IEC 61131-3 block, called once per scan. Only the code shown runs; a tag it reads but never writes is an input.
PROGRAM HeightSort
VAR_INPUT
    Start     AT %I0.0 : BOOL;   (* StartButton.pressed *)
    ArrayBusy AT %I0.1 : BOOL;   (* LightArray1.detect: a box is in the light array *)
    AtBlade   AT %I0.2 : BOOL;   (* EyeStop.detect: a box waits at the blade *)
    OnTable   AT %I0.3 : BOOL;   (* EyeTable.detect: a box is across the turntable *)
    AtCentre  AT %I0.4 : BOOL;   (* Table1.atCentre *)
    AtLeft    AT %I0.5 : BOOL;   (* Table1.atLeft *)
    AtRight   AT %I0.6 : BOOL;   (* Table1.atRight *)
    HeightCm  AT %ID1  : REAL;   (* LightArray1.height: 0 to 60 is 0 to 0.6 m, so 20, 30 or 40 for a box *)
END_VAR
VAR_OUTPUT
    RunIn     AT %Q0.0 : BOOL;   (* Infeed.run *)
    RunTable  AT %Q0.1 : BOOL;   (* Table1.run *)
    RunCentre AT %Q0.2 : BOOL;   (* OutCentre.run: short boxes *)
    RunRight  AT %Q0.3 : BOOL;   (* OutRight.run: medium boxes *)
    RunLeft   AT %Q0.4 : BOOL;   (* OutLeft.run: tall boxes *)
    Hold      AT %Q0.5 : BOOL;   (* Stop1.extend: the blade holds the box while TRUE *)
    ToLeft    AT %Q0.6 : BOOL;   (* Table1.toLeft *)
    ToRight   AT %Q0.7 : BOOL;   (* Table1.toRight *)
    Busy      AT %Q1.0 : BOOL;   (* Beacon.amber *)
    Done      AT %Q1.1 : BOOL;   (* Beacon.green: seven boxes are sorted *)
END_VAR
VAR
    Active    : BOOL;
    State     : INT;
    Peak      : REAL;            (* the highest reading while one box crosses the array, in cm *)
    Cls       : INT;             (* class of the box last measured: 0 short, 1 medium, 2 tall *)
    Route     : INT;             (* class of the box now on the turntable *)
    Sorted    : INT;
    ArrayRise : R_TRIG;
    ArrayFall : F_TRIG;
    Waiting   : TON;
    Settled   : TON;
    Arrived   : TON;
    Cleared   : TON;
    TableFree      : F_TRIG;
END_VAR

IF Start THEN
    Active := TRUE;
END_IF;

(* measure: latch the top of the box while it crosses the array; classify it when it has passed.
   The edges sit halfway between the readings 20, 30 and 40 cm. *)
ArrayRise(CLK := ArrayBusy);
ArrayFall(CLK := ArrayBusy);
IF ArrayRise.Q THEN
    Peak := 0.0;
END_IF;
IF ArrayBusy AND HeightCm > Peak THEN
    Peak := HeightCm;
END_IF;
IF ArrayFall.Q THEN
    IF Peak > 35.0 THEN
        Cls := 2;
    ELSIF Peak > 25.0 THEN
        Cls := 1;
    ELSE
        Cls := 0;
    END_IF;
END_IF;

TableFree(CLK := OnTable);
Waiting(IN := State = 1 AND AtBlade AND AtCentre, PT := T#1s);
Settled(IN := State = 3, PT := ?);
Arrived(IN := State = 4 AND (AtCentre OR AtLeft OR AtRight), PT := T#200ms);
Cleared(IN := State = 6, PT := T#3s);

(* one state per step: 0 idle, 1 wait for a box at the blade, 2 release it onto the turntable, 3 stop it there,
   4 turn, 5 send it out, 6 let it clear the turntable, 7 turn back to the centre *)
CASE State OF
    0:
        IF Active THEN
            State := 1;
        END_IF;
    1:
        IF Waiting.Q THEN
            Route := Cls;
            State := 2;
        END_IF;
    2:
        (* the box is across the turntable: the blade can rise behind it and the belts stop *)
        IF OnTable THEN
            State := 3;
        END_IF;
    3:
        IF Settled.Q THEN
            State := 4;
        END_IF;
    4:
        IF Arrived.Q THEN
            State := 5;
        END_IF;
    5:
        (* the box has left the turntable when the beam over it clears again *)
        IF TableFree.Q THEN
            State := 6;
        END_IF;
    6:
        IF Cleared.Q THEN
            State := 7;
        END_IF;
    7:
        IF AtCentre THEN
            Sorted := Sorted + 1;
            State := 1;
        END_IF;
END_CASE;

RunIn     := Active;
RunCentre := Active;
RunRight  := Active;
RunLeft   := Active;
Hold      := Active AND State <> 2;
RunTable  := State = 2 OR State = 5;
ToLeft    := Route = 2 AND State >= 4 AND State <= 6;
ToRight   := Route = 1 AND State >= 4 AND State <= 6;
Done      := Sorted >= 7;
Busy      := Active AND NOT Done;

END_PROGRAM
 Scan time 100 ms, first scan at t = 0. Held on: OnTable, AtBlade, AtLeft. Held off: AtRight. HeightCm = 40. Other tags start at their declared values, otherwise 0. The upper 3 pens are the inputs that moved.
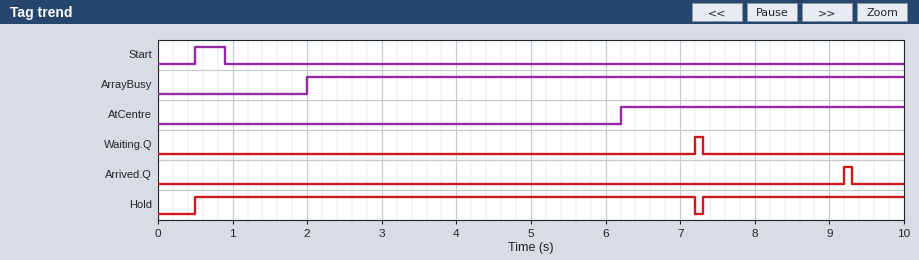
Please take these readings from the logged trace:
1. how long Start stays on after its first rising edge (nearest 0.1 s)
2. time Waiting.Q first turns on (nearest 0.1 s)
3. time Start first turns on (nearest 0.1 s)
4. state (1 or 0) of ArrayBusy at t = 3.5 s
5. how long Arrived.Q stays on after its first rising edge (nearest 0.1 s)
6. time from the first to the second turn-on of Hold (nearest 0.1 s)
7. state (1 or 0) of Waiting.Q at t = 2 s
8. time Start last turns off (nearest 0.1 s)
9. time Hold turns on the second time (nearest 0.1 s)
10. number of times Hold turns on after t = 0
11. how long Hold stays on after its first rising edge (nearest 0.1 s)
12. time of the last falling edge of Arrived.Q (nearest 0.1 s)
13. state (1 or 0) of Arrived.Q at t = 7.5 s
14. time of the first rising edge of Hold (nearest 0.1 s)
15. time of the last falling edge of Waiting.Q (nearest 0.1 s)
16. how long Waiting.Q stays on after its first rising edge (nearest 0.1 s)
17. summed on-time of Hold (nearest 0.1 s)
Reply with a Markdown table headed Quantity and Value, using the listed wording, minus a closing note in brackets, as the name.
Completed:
| Quantity | Value |
|---|---|
| how long Start stays on after its first rising edge | 0.4 s |
| time Waiting.Q first turns on | 7.2 s |
| time Start first turns on | 0.5 s |
| state (1 or 0) of ArrayBusy at t = 3.5 s | 1 |
| how long Arrived.Q stays on after its first rising edge | 0.1 s |
| time from the first to the second turn-on of Hold | 6.8 s |
| state (1 or 0) of Waiting.Q at t = 2 s | 0 |
| time Start last turns off | 0.9 s |
| time Hold turns on the second time | 7.3 s |
| number of times Hold turns on after t = 0 | 2 |
| how long Hold stays on after its first rising edge | 6.7 s |
| time of the last falling edge of Arrived.Q | 9.3 s |
| state (1 or 0) of Arrived.Q at t = 7.5 s | 0 |
| time of the first rising edge of Hold | 0.5 s |
| time of the last falling edge of Waiting.Q | 7.3 s |
| how long Waiting.Q stays on after its first rising edge | 0.1 s |
| summed on-time of Hold | 9.4 s |
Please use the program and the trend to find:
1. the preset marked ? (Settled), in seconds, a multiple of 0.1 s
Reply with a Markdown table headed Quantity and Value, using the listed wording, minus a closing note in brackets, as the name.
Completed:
| Quantity | Value |
|---|---|
| the preset marked ? (Settled), in seconds, a multiple of 0.1 s | 1.5 s |
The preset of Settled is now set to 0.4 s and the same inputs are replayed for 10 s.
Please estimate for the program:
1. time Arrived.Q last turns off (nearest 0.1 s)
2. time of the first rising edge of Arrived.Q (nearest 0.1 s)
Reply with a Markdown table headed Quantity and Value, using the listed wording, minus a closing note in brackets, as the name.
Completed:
| Quantity | Value |
|---|---|
| time Arrived.Q last turns off | 8.2 s |
| time of the first rising edge of Arrived.Q | 8.1 s |
